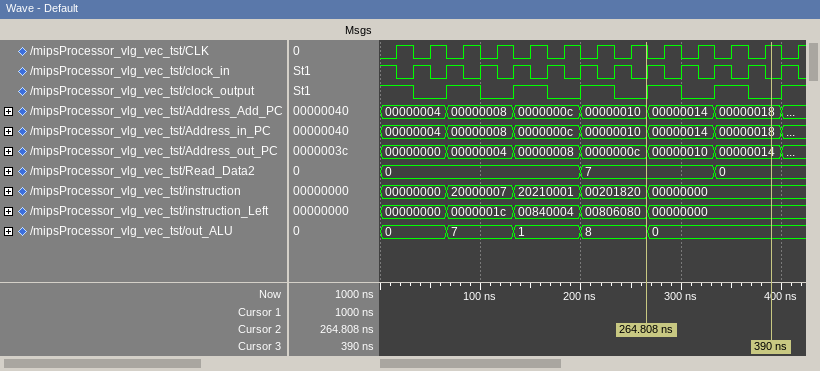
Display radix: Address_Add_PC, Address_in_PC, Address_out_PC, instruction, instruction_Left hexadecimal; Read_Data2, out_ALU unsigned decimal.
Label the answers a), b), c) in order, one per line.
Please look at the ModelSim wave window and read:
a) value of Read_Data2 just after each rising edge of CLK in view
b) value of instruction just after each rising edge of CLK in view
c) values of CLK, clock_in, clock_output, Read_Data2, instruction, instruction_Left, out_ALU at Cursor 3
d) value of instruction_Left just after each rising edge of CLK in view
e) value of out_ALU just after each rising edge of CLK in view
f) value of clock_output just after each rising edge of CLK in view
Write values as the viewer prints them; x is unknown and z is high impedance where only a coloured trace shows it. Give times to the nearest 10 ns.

a) 0, 0, 0, 0, 0, 0, 7, 7, 7, 7, 0, 0, 0
b) 00000000, 00000000, 20000007, 20000007, 20210001, 20210001, 00201820, 00201820, 00000000, 00000000, 00000000, 00000000, 00000000
c) CLK=1, clock_in=0, clock_output=0, Read_Data2=0, instruction=00000000, instruction_Left=00000000, out_ALU=0
d) 00000000, 00000000, 0000001c, 0000001c, 00840004, 00840004, 00806080, 00806080, 00000000, 00000000, 00000000, 00000000, 00000000
e) 0, 0, 7, 7, 1, 1, 8, 8, 0, 0, 0, 0, 0
f) 1 0 1 0 1 0 1 0 1 0 1 0 1
